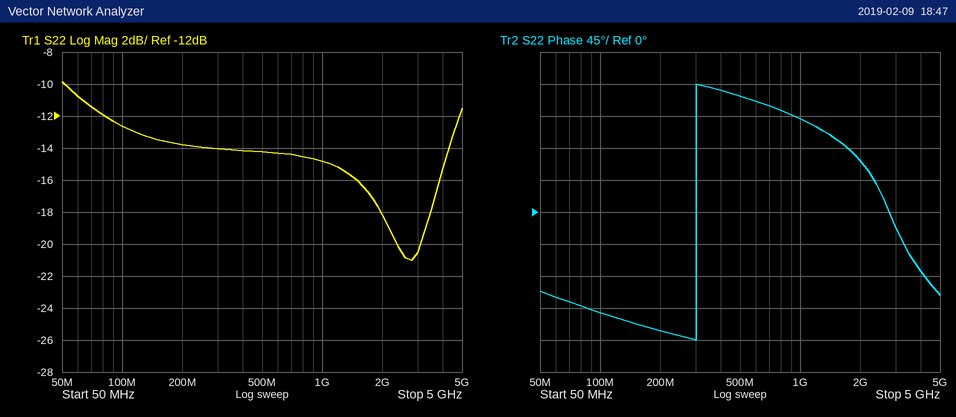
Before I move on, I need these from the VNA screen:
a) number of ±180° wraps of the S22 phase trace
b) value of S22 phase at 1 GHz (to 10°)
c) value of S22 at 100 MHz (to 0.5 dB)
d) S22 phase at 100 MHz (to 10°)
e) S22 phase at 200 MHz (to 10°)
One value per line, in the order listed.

1
130°
-12.5 dB
-140°
-170°
